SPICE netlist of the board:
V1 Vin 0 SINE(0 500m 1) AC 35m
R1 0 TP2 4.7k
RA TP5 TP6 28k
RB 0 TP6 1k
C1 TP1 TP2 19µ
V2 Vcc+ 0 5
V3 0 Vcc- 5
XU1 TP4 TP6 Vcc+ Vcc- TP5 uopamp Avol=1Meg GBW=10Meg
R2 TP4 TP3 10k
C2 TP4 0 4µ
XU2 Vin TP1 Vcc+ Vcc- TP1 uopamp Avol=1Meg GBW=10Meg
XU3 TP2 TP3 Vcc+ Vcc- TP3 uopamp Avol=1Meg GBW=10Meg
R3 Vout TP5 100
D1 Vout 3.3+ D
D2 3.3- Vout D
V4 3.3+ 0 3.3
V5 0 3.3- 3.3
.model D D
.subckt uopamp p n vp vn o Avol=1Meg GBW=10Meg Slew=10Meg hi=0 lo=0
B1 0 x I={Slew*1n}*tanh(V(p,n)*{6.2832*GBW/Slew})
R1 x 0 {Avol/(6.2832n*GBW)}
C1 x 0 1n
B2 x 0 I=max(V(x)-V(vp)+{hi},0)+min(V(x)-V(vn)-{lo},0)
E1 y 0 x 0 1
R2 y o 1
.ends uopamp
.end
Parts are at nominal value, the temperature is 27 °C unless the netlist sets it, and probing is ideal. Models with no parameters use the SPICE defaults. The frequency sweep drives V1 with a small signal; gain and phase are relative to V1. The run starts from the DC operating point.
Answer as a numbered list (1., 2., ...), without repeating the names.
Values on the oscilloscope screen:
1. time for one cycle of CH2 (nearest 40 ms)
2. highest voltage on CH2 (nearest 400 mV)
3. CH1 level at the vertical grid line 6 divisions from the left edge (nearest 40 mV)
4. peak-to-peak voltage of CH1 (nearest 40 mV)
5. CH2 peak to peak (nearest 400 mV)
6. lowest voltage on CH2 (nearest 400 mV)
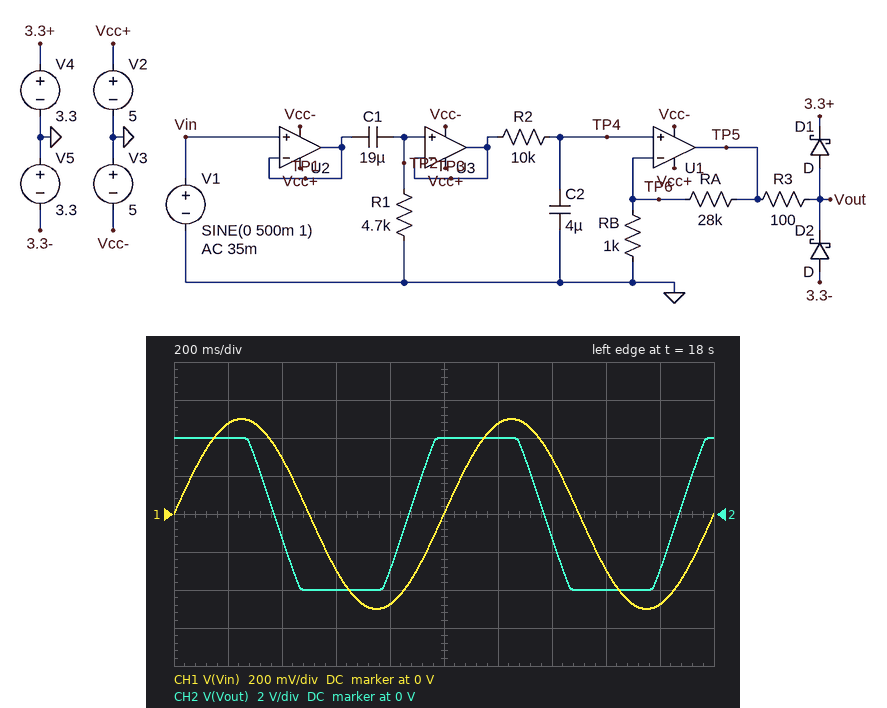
1. 1.00 s
2. 4.0 V
3. 480 mV
4. 1.00 V
5. 8.0 V
6. -4.0 V
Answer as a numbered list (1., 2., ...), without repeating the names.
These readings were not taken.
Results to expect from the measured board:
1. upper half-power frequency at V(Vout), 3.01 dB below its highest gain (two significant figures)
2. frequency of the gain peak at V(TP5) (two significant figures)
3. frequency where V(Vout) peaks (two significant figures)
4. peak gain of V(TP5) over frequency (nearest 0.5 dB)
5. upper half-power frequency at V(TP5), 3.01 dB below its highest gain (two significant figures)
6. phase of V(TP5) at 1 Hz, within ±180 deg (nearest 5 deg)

1. 6.8 Hz
2. 2.7 Hz
3. 2.7 Hz
4. 26.0 dB
5. 6.8 Hz
6. 45 deg
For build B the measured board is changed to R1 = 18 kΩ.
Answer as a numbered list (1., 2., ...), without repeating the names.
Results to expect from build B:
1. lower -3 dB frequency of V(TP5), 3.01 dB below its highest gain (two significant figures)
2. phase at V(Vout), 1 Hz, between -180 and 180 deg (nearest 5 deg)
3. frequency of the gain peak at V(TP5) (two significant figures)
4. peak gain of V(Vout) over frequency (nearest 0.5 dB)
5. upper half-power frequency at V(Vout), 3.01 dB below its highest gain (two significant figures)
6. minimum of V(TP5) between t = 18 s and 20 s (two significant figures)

1. 380 mHz
2. 10 deg
3. 1.4 Hz
4. 28.5 dB
5. 4.8 Hz
6. -5.0 V
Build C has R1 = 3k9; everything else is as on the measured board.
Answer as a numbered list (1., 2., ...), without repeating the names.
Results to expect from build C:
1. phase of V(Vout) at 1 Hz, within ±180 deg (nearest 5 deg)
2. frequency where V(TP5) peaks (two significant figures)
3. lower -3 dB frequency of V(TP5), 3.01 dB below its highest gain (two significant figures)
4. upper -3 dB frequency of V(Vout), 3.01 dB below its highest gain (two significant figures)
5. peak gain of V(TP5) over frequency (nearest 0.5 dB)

1. 50 deg
2. 2.9 Hz
3. 1.2 Hz
4. 7.3 Hz
5. 25.5 dB
